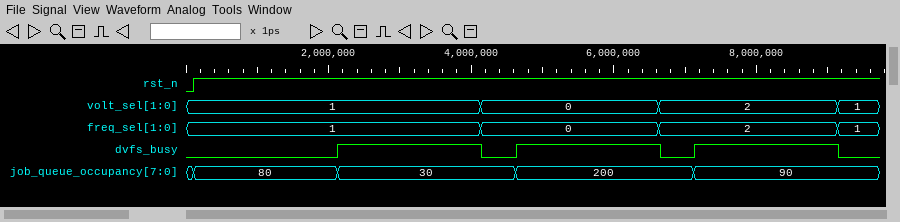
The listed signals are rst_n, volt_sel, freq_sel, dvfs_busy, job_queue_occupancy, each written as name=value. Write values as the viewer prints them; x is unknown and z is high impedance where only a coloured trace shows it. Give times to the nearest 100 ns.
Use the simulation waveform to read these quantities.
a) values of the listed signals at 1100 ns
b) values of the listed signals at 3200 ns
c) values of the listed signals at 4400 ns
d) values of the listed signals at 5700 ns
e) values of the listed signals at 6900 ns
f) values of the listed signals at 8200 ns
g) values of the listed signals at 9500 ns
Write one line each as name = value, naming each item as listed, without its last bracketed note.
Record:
values of the listed signals at 1100 ns = rst_n=1, volt_sel=1, freq_sel=1, dvfs_busy=0, job_queue_occupancy=80
values of the listed signals at 3200 ns = rst_n=1, volt_sel=1, freq_sel=1, dvfs_busy=1, job_queue_occupancy=30
values of the listed signals at 4400 ns = rst_n=1, volt_sel=0, freq_sel=0, dvfs_busy=0, job_queue_occupancy=30
values of the listed signals at 5700 ns = rst_n=1, volt_sel=0, freq_sel=0, dvfs_busy=1, job_queue_occupancy=200
values of the listed signals at 6900 ns = rst_n=1, volt_sel=2, freq_sel=2, dvfs_busy=0, job_queue_occupancy=200
values of the listed signals at 8200 ns = rst_n=1, volt_sel=2, freq_sel=2, dvfs_busy=1, job_queue_occupancy=90
values of the listed signals at 9500 ns = rst_n=1, volt_sel=1, freq_sel=1, dvfs_busy=0, job_queue_occupancy=90
